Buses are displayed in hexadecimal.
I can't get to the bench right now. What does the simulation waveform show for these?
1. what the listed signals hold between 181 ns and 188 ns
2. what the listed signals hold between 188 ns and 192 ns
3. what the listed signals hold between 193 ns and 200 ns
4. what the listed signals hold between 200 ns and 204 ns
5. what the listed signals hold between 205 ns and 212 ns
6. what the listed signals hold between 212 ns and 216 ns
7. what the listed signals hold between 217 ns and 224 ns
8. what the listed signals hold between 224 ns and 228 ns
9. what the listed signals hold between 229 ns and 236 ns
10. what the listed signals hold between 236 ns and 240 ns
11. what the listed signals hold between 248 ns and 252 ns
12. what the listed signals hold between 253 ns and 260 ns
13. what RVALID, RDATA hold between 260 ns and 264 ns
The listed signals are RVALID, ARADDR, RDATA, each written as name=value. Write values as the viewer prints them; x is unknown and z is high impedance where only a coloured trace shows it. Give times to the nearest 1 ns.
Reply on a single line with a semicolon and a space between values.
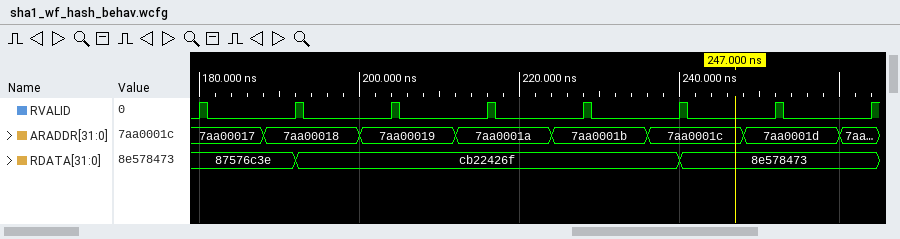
RVALID=0, ARADDR=7aa00017, RDATA=87576c3e; RVALID=0, ARADDR=7aa00018, RDATA=87576c3e; RVALID=0, ARADDR=7aa00018, RDATA=cb22426f; RVALID=0, ARADDR=7aa00019, RDATA=cb22426f; RVALID=0, ARADDR=7aa00019, RDATA=cb22426f; RVALID=0, ARADDR=7aa0001a, RDATA=cb22426f; RVALID=0, ARADDR=7aa0001a, RDATA=cb22426f; RVALID=0, ARADDR=7aa0001b, RDATA=cb22426f; RVALID=0, ARADDR=7aa0001b, RDATA=cb22426f; RVALID=0, ARADDR=7aa0001c, RDATA=cb22426f; RVALID=0, ARADDR=7aa0001d, RDATA=8e578473; RVALID=0, ARADDR=7aa0001d, RDATA=8e578473; RVALID=0, RDATA=8e578473
